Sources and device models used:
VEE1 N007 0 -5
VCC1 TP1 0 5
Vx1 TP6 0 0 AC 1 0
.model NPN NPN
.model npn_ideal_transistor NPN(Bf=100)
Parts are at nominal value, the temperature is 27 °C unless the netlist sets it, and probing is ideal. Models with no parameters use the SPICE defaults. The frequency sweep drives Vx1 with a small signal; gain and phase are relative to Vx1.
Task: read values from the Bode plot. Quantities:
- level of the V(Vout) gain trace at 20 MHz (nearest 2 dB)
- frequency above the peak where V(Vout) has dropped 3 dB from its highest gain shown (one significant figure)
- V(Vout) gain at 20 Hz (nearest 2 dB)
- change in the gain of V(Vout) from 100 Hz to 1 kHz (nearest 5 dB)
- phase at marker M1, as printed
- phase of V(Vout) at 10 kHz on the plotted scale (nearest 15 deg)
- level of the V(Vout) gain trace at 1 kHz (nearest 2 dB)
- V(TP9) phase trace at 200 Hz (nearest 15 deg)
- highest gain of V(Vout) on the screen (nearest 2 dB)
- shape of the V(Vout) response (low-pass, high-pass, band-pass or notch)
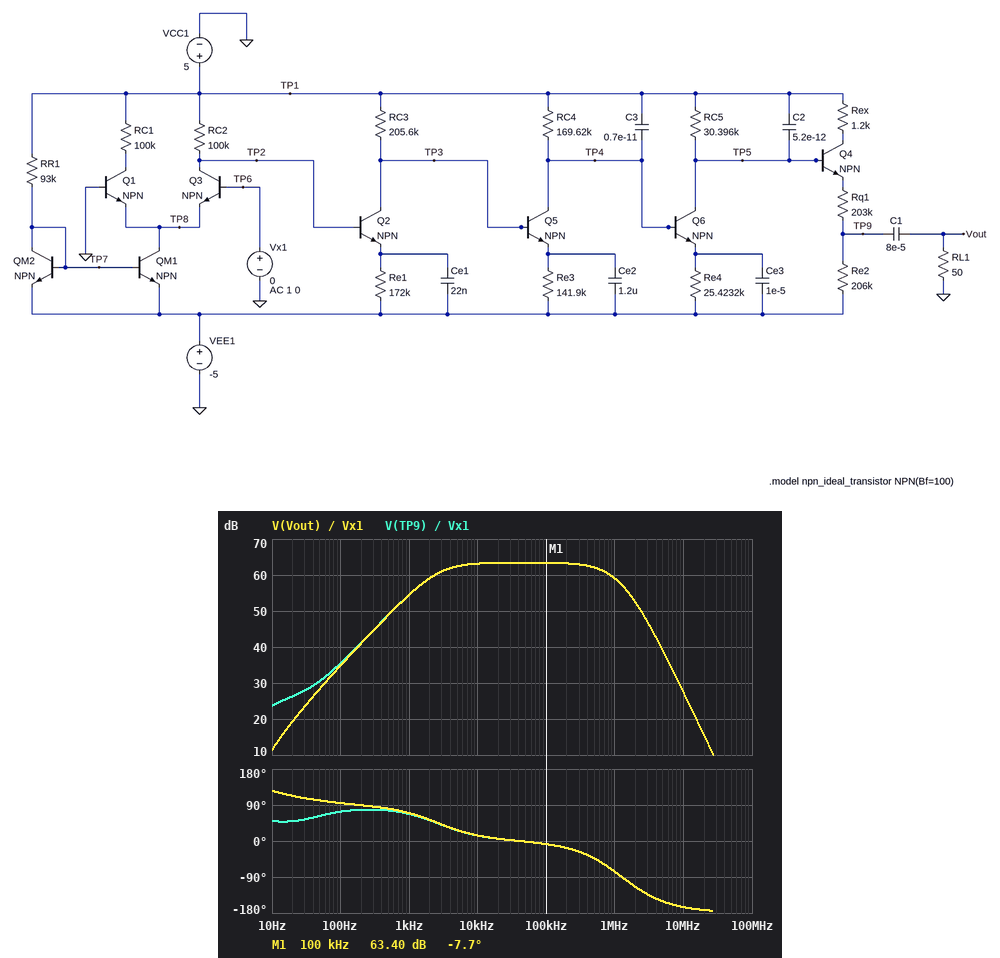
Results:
16 dB
800 kHz
20 dB
20 dB
-7.7 deg
15 deg
54 dB
75 deg
64 dB
band-pass
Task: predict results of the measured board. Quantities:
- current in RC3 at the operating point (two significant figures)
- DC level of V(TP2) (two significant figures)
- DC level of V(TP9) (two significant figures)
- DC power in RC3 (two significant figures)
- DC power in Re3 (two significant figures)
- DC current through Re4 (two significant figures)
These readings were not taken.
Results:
26 µA
130 mV
-2.8 V
140 µW
110 µW
170 µA
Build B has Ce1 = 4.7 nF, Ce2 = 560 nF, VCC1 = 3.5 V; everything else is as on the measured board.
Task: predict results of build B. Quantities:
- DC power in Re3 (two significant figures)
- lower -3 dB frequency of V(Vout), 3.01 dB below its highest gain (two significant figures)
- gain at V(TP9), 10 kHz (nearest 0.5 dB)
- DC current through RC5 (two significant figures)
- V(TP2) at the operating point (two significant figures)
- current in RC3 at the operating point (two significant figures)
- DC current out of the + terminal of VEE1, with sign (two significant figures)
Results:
78 µW
17 kHz
49.5 dB
140 µA
-560 mV
22 µA
-360 µA
